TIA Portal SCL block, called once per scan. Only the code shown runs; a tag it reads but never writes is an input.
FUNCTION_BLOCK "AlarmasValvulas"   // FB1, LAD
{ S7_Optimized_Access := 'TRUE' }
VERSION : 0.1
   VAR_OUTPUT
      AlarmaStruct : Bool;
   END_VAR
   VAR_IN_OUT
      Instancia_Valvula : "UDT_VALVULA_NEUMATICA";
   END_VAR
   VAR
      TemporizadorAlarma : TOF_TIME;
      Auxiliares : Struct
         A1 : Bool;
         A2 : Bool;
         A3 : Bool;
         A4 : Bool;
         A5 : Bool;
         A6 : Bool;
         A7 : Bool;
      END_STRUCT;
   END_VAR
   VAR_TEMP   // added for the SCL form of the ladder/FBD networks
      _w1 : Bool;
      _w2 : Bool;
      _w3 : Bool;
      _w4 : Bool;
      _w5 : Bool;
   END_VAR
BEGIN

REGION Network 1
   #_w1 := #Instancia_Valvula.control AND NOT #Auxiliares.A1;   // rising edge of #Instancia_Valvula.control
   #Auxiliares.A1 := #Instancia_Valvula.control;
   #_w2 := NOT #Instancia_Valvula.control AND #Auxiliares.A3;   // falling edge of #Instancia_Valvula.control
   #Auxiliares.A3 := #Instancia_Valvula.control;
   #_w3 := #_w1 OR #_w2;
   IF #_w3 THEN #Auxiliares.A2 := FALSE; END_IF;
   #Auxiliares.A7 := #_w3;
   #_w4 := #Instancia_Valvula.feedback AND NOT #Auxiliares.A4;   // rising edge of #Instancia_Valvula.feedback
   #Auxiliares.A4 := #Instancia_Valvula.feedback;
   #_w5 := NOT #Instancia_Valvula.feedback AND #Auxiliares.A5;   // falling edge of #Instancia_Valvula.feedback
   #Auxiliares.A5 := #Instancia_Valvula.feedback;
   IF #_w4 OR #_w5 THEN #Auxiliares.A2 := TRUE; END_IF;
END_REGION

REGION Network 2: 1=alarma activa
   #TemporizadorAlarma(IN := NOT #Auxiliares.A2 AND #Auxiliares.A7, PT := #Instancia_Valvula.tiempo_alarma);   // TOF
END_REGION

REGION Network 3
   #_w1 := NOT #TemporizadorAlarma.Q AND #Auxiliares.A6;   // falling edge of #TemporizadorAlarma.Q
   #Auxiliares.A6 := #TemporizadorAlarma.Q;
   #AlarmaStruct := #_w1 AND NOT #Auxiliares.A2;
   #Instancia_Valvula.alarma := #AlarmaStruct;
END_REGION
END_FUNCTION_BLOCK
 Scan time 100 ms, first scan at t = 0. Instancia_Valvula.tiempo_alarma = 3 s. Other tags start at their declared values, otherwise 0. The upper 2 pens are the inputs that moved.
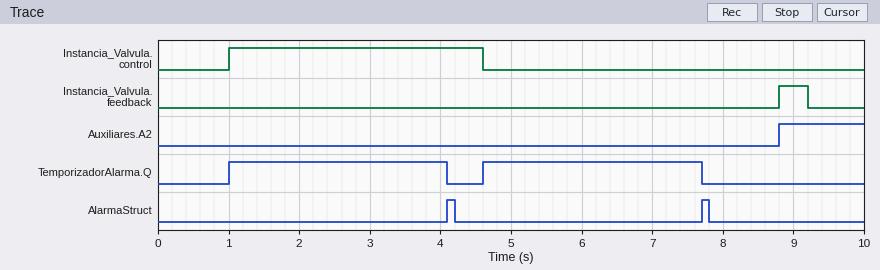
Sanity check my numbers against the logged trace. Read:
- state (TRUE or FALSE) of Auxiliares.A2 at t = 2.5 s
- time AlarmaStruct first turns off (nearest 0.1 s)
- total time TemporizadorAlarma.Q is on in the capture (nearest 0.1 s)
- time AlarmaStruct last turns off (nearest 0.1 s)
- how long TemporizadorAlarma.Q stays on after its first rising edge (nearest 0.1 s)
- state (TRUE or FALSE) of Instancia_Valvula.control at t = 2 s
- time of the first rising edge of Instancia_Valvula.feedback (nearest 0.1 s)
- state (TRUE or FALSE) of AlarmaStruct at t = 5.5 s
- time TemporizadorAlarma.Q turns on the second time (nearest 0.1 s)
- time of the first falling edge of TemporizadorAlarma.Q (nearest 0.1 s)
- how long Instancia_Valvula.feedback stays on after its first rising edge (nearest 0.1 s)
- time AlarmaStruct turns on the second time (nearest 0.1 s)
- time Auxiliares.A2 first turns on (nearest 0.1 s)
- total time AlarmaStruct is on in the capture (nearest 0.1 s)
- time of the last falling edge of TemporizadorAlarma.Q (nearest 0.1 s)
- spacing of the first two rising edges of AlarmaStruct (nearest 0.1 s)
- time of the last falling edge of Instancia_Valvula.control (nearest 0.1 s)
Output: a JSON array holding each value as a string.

["FALSE", "4.2 s", "6.2 s", "7.8 s", "3.1 s", "TRUE", "8.8 s", "FALSE", "4.6 s", "4.1 s", "0.4 s", "7.7 s", "8.8 s", "0.2 s", "7.7 s", "3.6 s", "4.6 s"]
